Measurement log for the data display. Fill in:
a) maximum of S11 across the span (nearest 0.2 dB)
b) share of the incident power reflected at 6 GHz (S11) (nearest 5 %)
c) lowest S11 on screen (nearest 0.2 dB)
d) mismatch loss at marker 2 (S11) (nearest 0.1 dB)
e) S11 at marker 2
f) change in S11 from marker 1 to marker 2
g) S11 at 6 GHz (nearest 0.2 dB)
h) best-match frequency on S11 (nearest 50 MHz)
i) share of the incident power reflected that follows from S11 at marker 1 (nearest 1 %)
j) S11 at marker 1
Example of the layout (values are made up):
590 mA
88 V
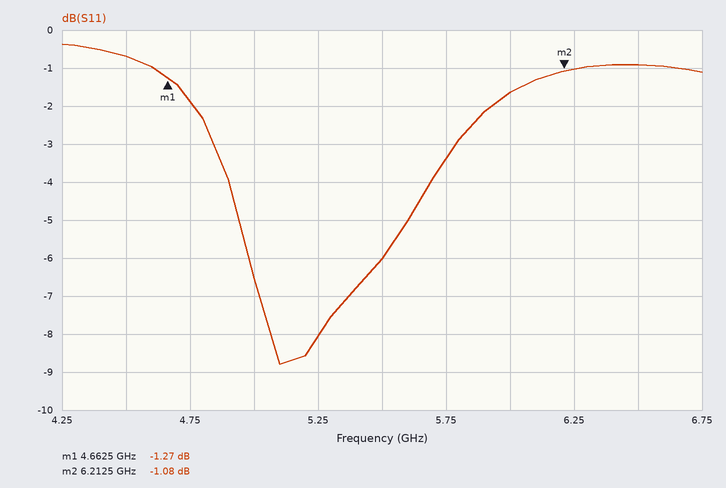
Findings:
-0.4 dB
70 %
-8.8 dB
6.6 dB
-1.08 dB
0.19 dB
-1.6 dB
5.10 GHz
75 %
-1.27 dB
